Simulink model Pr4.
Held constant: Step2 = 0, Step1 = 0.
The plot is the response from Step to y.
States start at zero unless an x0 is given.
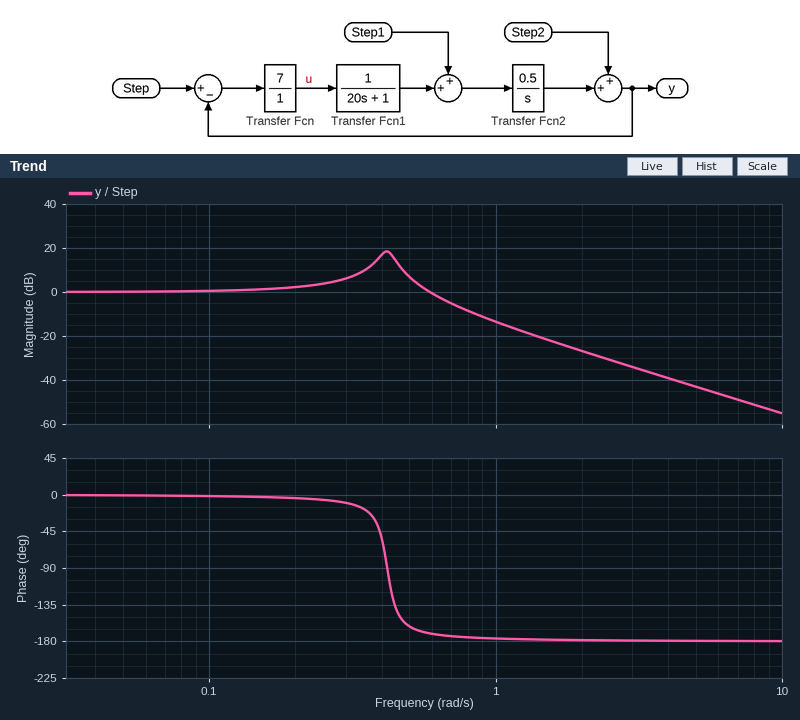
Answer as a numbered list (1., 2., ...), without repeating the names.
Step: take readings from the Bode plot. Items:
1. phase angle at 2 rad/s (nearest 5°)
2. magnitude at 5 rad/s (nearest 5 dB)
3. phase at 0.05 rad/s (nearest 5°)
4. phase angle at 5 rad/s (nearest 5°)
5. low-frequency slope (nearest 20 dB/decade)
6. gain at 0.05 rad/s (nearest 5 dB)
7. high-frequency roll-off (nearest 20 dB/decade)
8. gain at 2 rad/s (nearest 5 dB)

1. -180°
2. -45 dB
3. 0°
4. -180°
5. 0 dB/decade
6. 0 dB
7. -40 dB/decade
8. -25 dB
